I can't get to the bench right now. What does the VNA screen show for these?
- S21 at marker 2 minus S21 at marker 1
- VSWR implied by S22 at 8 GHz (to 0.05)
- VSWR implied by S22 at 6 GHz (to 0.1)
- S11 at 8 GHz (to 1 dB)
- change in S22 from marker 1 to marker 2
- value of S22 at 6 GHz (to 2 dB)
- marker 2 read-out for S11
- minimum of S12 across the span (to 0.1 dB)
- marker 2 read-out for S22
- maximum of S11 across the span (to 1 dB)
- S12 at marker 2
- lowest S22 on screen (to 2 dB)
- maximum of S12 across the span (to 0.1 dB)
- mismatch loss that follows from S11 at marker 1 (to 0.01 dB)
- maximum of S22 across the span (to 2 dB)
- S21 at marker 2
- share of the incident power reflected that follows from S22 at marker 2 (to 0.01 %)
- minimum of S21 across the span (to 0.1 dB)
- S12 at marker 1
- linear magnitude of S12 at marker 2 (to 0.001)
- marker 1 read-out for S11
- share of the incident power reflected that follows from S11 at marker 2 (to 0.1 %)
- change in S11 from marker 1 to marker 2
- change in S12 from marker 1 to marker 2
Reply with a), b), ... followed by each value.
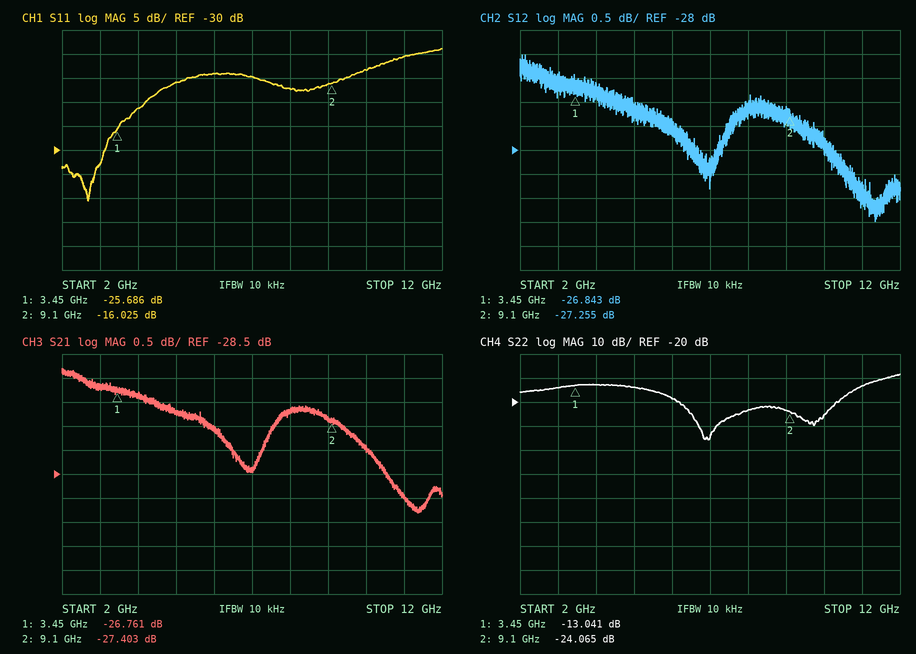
a) -0.642 dB
b) 1.15
c) 1.3
d) -17 dB
e) -11.024 dB
f) -18 dB
g) -16.025 dB
h) -29.5 dB
i) -24.065 dB
j) -9 dB
k) -27.255 dB
l) -36 dB
m) -26.0 dB
n) 0.01 dB
o) -8 dB
p) -27.403 dB
q) 0.39 %
r) -29.3 dB
s) -26.843 dB
t) 0.043
u) -25.686 dB
v) 2.5 %
w) 9.661 dB
x) -0.412 dB
